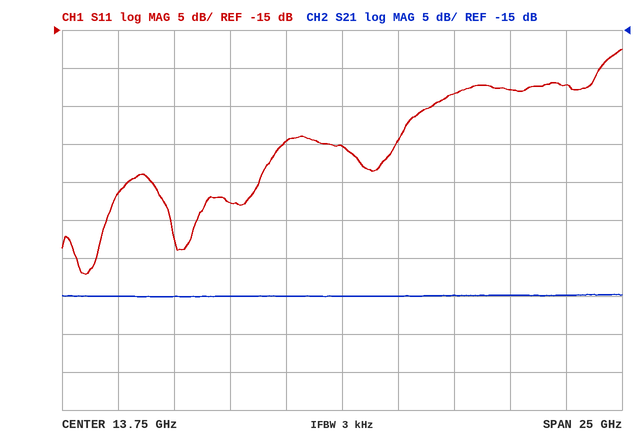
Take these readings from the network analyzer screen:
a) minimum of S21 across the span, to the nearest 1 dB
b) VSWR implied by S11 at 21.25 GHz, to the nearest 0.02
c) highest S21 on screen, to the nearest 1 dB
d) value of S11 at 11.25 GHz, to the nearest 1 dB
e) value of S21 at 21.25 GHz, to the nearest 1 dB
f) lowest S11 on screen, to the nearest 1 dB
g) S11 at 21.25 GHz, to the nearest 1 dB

-50 dB
1.16
-50 dB
-30 dB
-50 dB
-47 dB
-23 dB
